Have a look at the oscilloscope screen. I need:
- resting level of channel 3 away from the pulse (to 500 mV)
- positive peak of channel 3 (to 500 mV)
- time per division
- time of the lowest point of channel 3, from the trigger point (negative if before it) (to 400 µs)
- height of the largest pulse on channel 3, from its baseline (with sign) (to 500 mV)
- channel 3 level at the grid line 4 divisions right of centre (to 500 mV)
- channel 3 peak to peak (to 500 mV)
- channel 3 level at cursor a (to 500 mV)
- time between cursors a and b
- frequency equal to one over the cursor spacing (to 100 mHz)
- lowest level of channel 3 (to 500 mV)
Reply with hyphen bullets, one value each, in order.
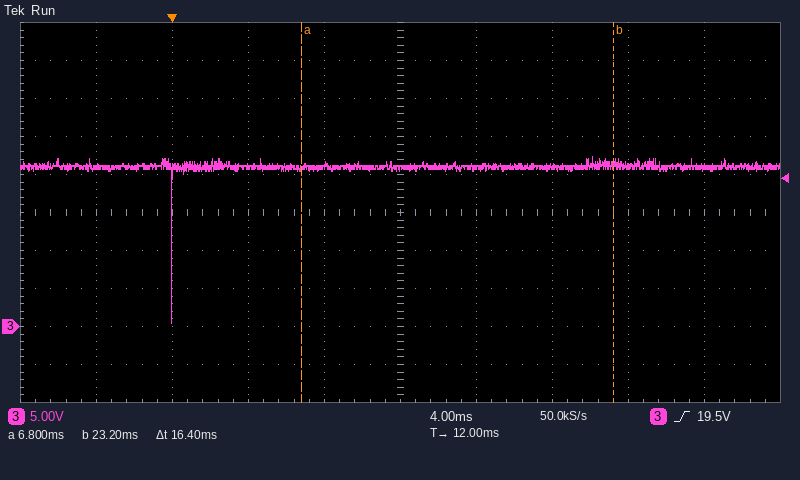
- 21.0 V
- 22.5 V
- 4 ms
- 0.0 ms
- -20.5 V
- 21.0 V
- 22.0 V
- 21.0 V
- 16.4 ms
- 61.0 Hz
- 500 mV
